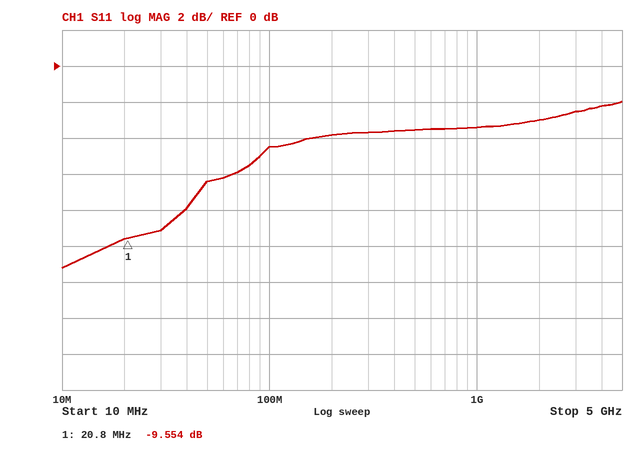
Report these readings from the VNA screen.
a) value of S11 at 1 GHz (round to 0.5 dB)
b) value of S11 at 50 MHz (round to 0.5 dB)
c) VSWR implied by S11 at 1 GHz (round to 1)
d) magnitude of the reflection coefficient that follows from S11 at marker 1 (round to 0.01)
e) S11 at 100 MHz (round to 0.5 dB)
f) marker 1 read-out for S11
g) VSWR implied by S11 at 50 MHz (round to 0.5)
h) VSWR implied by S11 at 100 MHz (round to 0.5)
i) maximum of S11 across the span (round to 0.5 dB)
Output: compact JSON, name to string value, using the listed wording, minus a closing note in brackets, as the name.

{"value of S11 at 1 GHz": "-3.5 dB", "value of S11 at 50 MHz": "-6.5 dB", "VSWR implied by S11 at 1 GHz": "5", "magnitude of the reflection coefficient that follows from S11 at marker 1": "0.33", "S11 at 100 MHz": "-4.5 dB", "marker 1 read-out for S11": "-9.554 dB", "VSWR implied by S11 at 50 MHz": "3.0", "VSWR implied by S11 at 100 MHz": "4.0", "maximum of S11 across the span": "-2.0 dB"}
